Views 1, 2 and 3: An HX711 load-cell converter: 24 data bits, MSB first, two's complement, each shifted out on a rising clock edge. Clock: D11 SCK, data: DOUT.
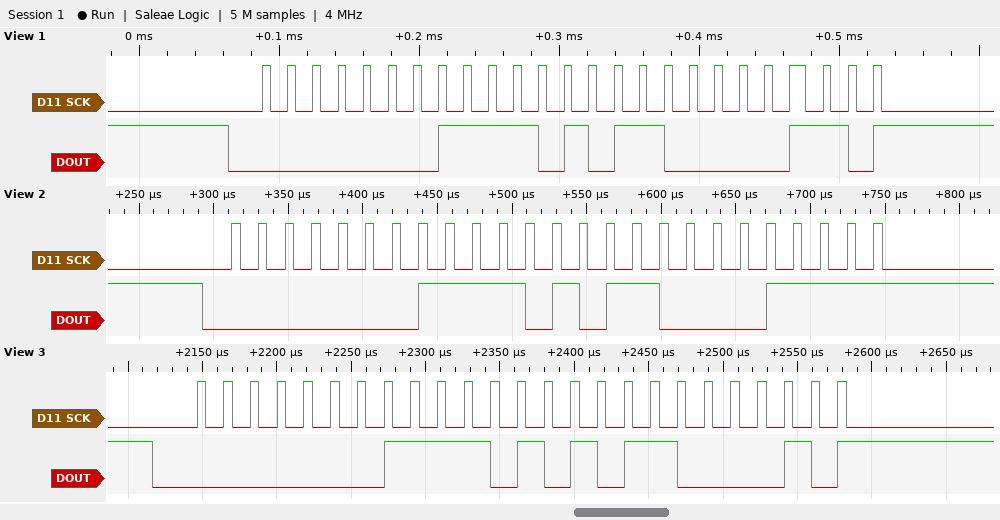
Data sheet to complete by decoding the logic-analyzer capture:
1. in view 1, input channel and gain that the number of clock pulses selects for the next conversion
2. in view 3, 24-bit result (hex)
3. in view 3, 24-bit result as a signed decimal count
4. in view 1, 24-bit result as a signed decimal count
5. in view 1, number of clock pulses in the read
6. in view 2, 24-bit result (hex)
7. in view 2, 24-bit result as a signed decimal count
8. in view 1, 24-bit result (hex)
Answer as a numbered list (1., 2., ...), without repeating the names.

1. channel A, gain 128
2. 0x01EAC2
3. 125634
4. 125702
5. 25
6. 0x01EB0F
7. 125711
8. 0x01EB06
